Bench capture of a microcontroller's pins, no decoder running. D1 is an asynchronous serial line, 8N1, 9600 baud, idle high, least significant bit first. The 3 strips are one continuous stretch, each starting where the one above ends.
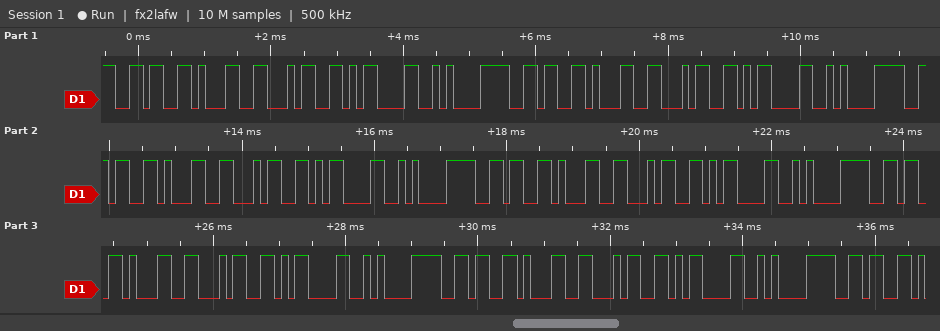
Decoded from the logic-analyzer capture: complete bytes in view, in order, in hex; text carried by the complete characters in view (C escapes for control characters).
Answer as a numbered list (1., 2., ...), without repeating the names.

1. 0x36 0x31 0x34 0x0D 0x0A 0x36 0x31 0x34 0x0D 0x0A 0x36 0x31 0x34 0x0D 0x0A 0x36 0x31 0x34 0x0D 0x0A 0x36 0x31 0x34 0x0D 0x0A 0x36 0x31 0x34 0x0D 0x0A 0x36
2. "614\r\n614\r\n614\r\n614\r\n614\r\n614\r\n6"
